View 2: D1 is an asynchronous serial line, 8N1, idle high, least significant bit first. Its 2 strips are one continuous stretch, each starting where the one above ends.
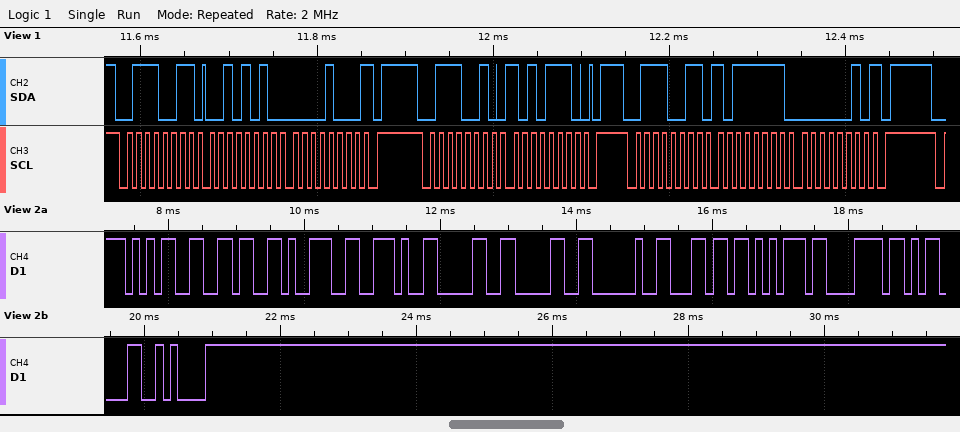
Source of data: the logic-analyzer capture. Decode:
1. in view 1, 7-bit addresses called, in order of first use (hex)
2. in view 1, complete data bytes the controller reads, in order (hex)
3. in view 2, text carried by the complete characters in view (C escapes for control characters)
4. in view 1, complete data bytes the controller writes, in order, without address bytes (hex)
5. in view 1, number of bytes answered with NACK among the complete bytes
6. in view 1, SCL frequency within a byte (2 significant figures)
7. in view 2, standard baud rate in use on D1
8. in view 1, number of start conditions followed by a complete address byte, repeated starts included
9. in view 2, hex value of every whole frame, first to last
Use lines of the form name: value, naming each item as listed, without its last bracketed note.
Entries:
in view 1, 7-bit addresses called, in order of first use: 0x39
in view 1, complete data bytes the controller reads, in order: 2A 08 BF 02
in view 2, text carried by the complete characters in view: "569.00 lux\r\n"
in view 1, complete data bytes the controller writes, in order, without address bytes: AE
in view 1, number of bytes answered with NACK among the complete bytes: 2
in view 1, SCL frequency within a byte: 100 kHz
in view 2, standard baud rate in use on D1: 9600 baud
in view 1, number of start conditions followed by a complete address byte, repeated starts included: 3
in view 2, hex value of every whole frame, first to last: 0x35 0x36 0x39 0x2E 0x30 0x30 0x20 0x6C 0x75 0x78 0x0D 0x0A
